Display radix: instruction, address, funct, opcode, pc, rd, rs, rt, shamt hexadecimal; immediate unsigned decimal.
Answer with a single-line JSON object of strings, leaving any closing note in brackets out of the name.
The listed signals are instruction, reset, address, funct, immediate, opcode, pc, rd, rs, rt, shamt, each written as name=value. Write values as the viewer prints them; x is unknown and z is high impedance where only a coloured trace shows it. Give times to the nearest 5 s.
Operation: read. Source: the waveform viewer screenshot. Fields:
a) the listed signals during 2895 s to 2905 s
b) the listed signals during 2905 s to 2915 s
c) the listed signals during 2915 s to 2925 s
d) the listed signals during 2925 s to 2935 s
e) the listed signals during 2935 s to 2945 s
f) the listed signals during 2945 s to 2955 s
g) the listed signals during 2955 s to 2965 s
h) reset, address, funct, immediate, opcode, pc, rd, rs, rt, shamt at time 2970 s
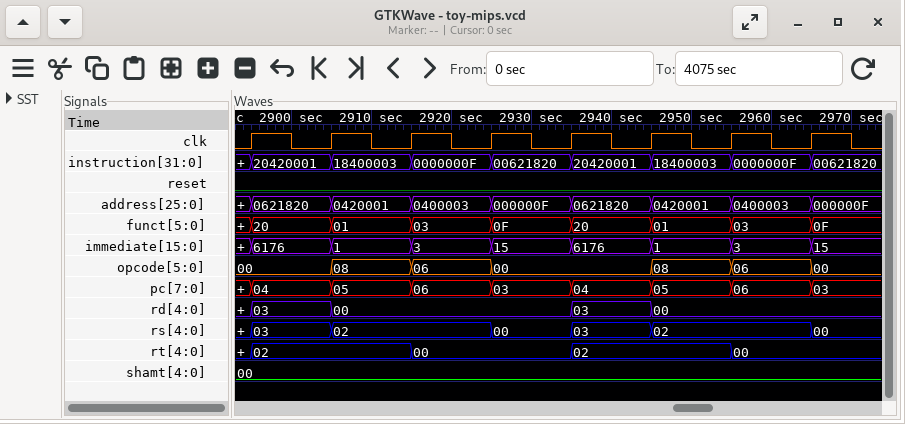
{"the listed signals during 2895 s to 2905 s": "instruction=20420001, reset=0, address=0621820, funct=20, immediate=6176, opcode=00, pc=04, rd=03, rs=03, rt=02, shamt=00", "the listed signals during 2905 s to 2915 s": "instruction=18400003, reset=0, address=0420001, funct=01, immediate=1, opcode=08, pc=05, rd=00, rs=02, rt=02, shamt=00", "the listed signals during 2915 s to 2925 s": "instruction=0000000F, reset=0, address=0400003, funct=03, immediate=3, opcode=06, pc=06, rd=00, rs=02, rt=00, shamt=00", "the listed signals during 2925 s to 2935 s": "instruction=00621820, reset=0, address=000000F, funct=0F, immediate=15, opcode=00, pc=03, rd=00, rs=00, rt=00, shamt=00", "the listed signals during 2935 s to 2945 s": "instruction=20420001, reset=0, address=0621820, funct=20, immediate=6176, opcode=00, pc=04, rd=03, rs=03, rt=02, shamt=00", "the listed signals during 2945 s to 2955 s": "instruction=18400003, reset=0, address=0420001, funct=01, immediate=1, opcode=08, pc=05, rd=00, rs=02, rt=02, shamt=00", "the listed signals during 2955 s to 2965 s": "instruction=0000000F, reset=0, address=0400003, funct=03, immediate=3, opcode=06, pc=06, rd=00, rs=02, rt=00, shamt=00", "reset, address, funct, immediate, opcode, pc, rd, rs, rt, shamt at time 2970 s": "reset=0, address=000000F, funct=0F, immediate=15, opcode=00, pc=03, rd=00, rs=00, rt=00, shamt=00"}
